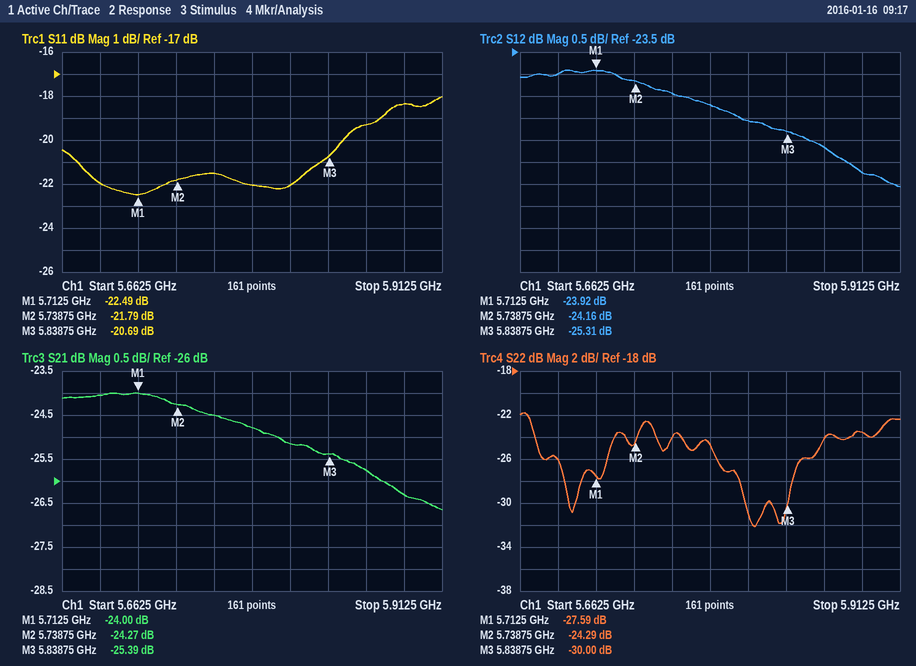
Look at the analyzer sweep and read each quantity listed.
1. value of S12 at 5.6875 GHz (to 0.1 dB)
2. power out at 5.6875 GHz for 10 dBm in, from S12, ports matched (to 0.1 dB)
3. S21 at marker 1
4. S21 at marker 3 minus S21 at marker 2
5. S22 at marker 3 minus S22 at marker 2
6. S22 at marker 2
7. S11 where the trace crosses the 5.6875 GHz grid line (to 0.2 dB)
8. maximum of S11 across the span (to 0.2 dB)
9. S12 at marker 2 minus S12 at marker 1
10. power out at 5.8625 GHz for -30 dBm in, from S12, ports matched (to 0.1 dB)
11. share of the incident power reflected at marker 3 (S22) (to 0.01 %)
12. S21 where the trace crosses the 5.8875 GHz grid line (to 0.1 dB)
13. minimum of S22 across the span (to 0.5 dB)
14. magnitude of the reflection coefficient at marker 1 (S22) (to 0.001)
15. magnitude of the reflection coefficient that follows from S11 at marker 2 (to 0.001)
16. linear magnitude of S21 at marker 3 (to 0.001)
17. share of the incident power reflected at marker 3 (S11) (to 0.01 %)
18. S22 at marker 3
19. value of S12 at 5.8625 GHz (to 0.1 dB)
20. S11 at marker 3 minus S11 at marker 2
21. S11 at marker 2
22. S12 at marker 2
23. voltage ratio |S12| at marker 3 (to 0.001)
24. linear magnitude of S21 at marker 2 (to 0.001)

-24.0 dB
-14.0 dBm
-24.00 dB
-1.12 dB
-5.71 dB
-24.29 dB
-22.0 dB
-18.0 dB
-0.24 dB
-55.7 dBm
0.10 %
-26.3 dB
-32.0 dB
0.042
0.081
0.054
0.85 %
-30.00 dB
-25.7 dB
1.10 dB
-21.79 dB
-24.16 dB
0.054
0.061
